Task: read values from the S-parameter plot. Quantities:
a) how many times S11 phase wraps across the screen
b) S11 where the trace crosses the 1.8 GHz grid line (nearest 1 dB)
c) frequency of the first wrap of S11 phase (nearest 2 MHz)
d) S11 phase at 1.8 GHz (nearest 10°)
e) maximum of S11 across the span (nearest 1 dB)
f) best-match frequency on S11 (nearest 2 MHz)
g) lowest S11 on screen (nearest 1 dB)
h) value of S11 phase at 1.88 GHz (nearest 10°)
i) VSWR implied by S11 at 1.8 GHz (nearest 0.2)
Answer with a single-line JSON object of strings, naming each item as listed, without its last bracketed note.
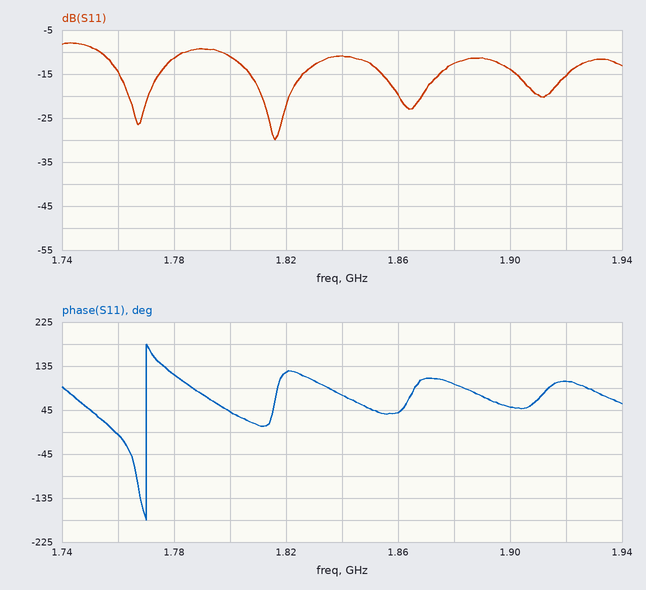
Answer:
{"how many times S11 phase wraps across the screen": "1", "S11 where the trace crosses the 1.8 GHz grid line": "-11 dB", "frequency of the first wrap of S11 phase": "1.770 GHz", "S11 phase at 1.8 GHz": "40°", "maximum of S11 across the span": "-8 dB", "best-match frequency on S11": "1.816 GHz", "lowest S11 on screen": "-30 dB", "value of S11 phase at 1.88 GHz": "100°", "VSWR implied by S11 at 1.8 GHz": "1.8"}
